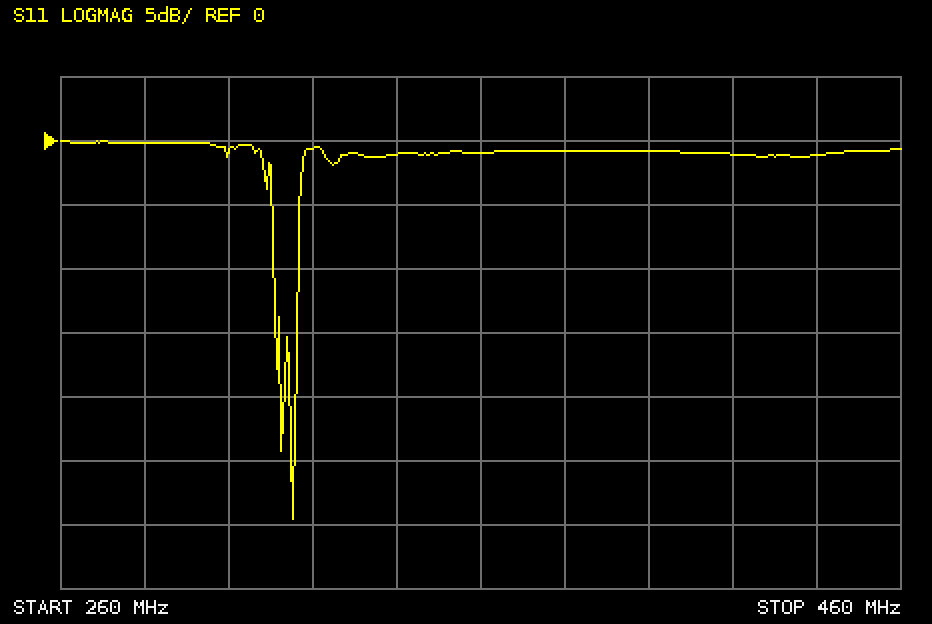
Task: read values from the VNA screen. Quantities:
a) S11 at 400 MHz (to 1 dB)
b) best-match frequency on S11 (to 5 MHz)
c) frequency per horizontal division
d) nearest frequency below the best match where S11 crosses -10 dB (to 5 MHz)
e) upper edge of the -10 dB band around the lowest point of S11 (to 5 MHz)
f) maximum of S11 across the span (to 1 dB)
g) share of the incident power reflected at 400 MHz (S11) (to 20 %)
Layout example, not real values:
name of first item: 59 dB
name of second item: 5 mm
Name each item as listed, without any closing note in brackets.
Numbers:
S11 at 400 MHz: -1 dB
best-match frequency on S11: 315 MHz
frequency per horizontal division: 20 MHz
nearest frequency below the best match where S11 crosses -10 dB: 310 MHz
upper edge of the -10 dB band around the lowest point of S11: 315 MHz
maximum of S11 across the span: 0 dB
share of the incident power reflected at 400 MHz (S11): 80 %
